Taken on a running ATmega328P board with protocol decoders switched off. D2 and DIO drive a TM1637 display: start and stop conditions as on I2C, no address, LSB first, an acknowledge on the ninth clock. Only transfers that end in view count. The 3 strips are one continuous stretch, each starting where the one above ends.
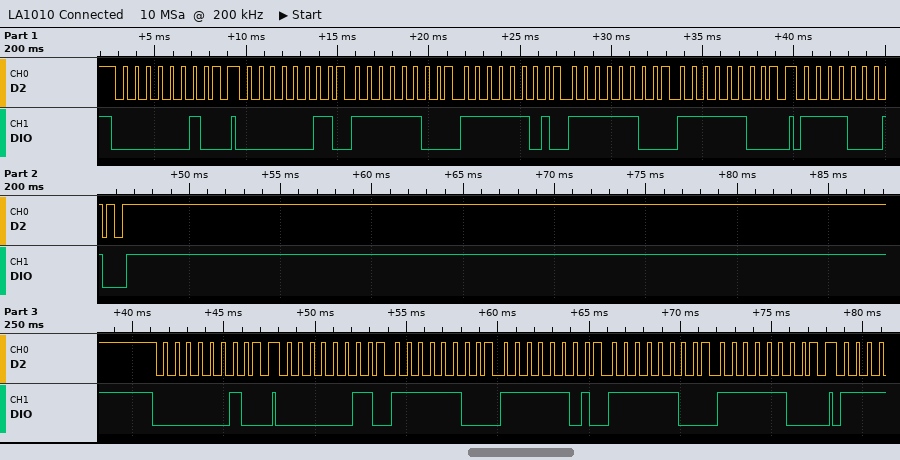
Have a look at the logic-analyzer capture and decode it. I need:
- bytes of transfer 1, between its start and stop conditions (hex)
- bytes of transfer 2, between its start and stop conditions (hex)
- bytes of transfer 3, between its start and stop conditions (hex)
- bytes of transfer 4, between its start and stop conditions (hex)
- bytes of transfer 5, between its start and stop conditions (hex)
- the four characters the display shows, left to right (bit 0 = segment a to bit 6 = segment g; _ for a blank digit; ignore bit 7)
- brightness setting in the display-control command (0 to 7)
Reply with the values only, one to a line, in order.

40
C0 3F BF 3F 3F
8F
40
C0 3F BF 3F 3F
0000
7
